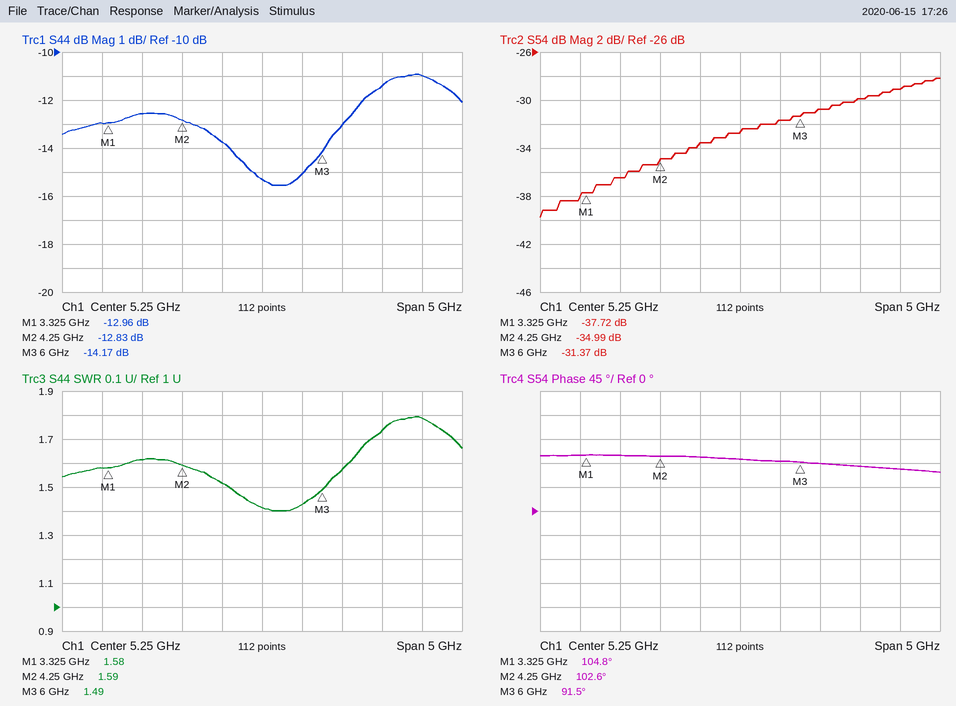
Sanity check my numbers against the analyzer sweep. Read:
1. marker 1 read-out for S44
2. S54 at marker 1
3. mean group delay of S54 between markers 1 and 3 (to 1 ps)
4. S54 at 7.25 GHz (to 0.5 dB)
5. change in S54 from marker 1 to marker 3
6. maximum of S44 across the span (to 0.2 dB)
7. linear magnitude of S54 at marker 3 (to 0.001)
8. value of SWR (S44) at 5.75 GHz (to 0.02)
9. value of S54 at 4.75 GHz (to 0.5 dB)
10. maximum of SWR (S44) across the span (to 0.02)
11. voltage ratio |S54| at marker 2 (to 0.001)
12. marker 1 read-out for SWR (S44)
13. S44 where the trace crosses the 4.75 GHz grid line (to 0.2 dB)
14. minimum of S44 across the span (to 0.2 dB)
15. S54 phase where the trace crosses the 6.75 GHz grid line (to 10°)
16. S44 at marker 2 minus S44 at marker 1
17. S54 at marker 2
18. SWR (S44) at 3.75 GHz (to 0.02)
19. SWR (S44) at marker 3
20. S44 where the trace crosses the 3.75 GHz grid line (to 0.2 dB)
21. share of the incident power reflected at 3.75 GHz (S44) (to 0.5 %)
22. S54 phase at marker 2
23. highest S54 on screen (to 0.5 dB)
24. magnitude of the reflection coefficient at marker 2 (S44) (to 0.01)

-12.96 dB
-37.72 dB
14 ps
-29.0 dB
6.35 dB
-11.0 dB
0.027
1.42
-33.5 dB
1.80
0.018
1.58
-13.8 dB
-15.6 dB
80°
0.13 dB
-34.99 dB
1.62
1.49
-12.6 dB
5.5 %
102.6°
-28.0 dB
0.23
